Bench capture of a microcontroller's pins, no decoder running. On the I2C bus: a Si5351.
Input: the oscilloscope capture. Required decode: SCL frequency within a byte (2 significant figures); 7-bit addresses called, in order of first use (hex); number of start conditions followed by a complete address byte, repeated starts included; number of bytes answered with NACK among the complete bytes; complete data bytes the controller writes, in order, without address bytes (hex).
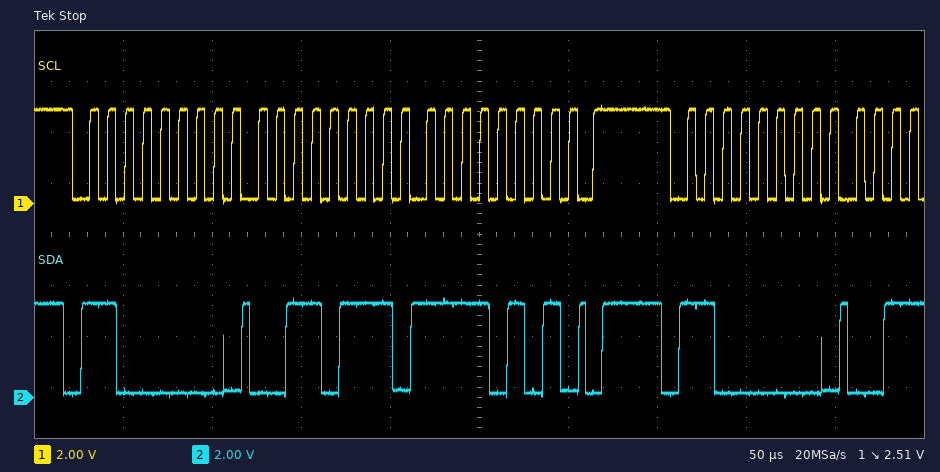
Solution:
100 kHz
0x60
2
0
37 F5
